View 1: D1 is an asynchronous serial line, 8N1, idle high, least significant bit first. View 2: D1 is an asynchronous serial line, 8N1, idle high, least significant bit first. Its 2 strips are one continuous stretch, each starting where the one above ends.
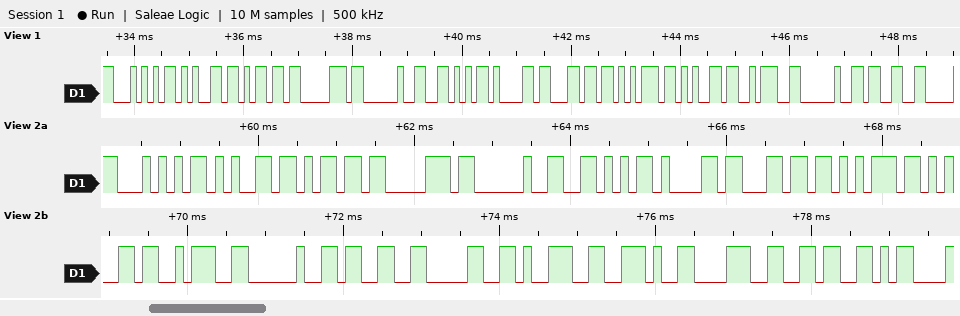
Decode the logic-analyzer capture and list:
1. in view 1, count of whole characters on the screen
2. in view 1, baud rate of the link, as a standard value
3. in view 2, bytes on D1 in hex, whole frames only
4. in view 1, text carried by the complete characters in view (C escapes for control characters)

13
9600 baud
0x54 0x65 0x6D 0x70 0x20 0x56 0x61 0x6C 0x75 0x65 0x3A 0x20 0x33 0x30 0x39 0x2E 0x38 0x36 0x0D
"Temp Value: 3"
